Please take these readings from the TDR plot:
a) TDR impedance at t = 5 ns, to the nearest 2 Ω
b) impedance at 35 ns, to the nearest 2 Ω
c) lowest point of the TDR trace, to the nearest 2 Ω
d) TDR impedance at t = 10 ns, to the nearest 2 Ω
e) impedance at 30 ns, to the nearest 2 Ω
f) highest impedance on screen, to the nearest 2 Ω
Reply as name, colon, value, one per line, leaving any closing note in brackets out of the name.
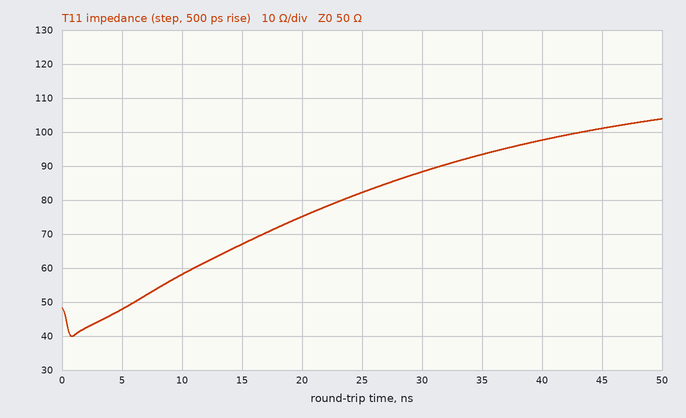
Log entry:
TDR impedance at t = 5 ns, to the nearest 2 Ω: 48 Ω
impedance at 35 ns, to the nearest 2 Ω: 94 Ω
lowest point of the TDR trace, to the nearest 2 Ω: 40 Ω
TDR impedance at t = 10 ns, to the nearest 2 Ω: 58 Ω
impedance at 30 ns, to the nearest 2 Ω: 88 Ω
highest impedance on screen, to the nearest 2 Ω: 104 Ω
